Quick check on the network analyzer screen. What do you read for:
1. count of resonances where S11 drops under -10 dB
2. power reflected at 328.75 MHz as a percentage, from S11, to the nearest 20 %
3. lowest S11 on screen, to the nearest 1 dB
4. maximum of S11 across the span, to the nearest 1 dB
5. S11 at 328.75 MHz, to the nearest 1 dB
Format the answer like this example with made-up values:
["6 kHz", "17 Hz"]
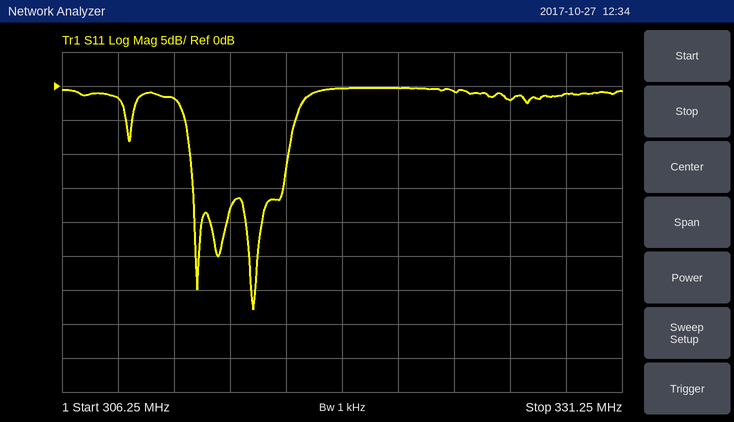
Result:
["3", "80 %", "-33 dB", "0 dB", "-1 dB"]
